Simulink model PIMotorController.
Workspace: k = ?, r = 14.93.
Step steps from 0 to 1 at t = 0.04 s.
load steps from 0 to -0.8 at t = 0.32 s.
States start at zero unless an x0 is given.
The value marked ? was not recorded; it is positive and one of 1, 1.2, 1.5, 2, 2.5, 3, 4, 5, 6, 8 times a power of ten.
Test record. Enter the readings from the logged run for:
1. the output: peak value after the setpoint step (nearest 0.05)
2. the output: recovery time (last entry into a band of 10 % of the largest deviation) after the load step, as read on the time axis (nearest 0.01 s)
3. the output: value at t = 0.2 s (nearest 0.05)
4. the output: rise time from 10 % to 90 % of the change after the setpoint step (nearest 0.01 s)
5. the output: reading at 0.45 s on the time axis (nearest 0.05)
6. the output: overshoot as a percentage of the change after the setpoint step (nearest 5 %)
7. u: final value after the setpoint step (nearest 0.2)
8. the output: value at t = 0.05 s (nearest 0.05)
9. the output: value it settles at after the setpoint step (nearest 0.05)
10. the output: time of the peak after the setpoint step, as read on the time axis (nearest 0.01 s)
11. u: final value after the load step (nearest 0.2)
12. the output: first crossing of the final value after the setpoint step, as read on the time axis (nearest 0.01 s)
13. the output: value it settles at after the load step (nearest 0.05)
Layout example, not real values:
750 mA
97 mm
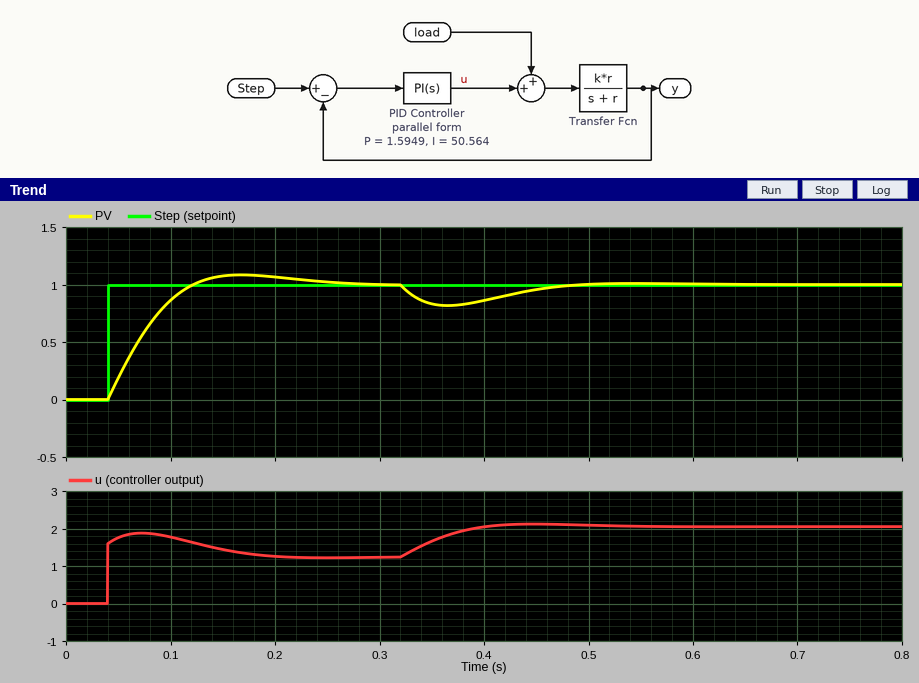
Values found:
1.10
0.47 s
1.05
0.06 s
0.95
10 %
1.2
0.20
1.00
0.17 s
2.0
0.12 s
1.00
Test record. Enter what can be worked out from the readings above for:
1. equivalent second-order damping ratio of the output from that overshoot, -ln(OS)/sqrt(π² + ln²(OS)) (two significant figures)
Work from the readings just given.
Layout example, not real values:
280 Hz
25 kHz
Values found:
0.59
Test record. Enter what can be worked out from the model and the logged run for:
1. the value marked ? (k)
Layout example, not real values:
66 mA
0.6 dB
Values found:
0.8
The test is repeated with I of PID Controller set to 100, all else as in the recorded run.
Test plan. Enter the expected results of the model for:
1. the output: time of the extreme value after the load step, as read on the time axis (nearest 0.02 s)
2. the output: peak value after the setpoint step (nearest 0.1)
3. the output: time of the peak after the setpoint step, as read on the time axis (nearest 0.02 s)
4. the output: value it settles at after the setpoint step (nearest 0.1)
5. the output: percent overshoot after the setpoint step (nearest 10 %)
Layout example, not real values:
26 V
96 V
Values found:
0.36 s
1.2
0.12 s
1.0
20 %
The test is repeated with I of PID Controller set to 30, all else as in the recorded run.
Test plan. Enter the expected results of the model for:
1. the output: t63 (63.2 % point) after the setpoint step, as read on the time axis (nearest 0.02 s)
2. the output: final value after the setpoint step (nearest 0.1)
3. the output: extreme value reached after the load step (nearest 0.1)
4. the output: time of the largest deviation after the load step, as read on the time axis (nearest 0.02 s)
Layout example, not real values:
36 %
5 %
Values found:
0.08 s
1.0
0.8
0.38 s
